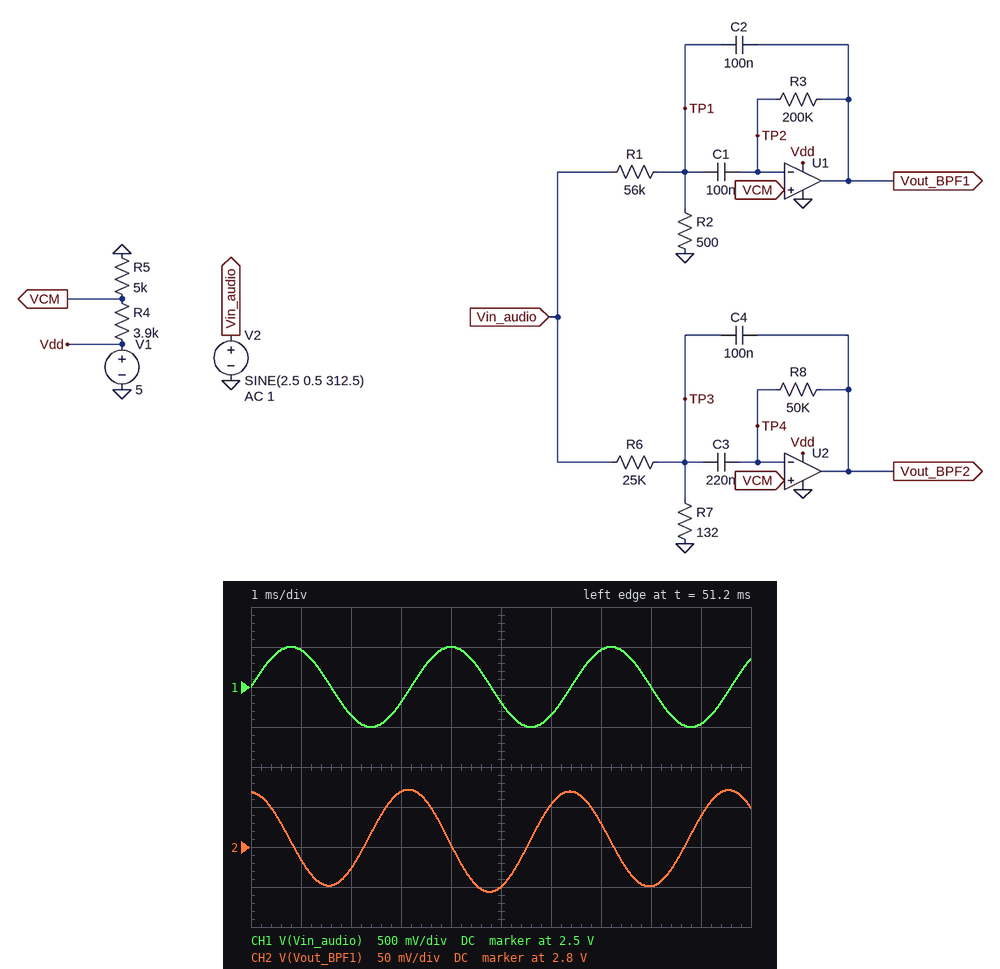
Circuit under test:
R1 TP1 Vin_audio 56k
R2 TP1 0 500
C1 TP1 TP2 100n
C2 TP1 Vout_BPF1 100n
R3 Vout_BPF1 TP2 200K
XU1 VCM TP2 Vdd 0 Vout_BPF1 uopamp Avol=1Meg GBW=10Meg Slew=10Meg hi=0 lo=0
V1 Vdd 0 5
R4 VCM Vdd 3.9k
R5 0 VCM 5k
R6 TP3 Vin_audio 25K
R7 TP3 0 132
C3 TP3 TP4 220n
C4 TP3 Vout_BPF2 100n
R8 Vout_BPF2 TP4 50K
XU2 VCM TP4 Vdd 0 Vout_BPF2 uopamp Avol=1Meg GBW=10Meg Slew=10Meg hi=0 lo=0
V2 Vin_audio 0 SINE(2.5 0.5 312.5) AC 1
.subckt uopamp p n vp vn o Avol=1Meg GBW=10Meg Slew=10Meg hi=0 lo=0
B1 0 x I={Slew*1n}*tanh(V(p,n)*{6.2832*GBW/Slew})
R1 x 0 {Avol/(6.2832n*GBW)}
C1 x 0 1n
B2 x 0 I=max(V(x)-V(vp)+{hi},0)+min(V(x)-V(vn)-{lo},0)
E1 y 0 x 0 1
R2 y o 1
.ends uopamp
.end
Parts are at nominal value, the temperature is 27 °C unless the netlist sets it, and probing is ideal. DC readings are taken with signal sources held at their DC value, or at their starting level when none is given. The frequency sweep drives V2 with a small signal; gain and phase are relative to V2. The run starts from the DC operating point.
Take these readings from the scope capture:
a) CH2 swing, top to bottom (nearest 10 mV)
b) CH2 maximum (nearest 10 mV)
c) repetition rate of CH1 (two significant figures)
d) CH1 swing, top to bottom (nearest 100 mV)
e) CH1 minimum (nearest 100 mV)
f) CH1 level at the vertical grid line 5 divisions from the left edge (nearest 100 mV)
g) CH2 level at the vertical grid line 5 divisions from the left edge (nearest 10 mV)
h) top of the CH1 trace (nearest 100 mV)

130 mV
2.87 V
310 Hz
1.0 V
2.0 V
2.3 V
2.75 V
3.0 V
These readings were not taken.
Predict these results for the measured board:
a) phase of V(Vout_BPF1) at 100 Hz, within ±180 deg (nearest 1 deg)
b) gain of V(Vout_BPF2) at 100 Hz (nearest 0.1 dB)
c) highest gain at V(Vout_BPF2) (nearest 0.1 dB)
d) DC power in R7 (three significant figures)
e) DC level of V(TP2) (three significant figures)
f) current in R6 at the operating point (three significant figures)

-96 deg
-28.3 dB
2.8 dB
1.31 µW
2.81 V
99.5 µA
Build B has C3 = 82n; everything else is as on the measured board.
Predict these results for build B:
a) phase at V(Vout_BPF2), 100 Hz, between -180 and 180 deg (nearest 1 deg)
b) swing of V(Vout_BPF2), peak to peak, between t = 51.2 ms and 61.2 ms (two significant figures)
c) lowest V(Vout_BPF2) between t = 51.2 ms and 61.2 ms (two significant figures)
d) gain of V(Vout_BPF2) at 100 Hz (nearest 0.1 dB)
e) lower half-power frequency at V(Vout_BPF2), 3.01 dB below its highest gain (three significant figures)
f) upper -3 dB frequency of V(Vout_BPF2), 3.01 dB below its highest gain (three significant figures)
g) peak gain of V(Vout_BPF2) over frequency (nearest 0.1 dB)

-91 deg
53 mV
2.8 V
-37.2 dB
651 Hz
722 Hz
-0.9 dB
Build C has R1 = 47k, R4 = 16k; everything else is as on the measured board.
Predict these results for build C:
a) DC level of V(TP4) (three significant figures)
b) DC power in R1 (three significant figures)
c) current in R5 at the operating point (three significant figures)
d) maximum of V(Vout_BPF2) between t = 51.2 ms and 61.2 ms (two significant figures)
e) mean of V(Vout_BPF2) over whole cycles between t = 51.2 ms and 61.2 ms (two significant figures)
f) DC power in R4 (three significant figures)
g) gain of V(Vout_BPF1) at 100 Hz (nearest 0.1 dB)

1.19 V
130 µW
238 µA
1.3 V
1.2 V
907 µW
-13.3 dB
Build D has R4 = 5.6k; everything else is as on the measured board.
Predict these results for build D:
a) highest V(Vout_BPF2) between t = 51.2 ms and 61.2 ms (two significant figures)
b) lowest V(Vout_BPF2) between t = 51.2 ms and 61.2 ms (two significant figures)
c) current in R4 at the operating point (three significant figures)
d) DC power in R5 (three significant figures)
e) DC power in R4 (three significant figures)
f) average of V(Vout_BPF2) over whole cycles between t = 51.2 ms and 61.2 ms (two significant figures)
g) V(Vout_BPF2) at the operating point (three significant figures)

2.5 V
2.2 V
472 µA
1.11 mW
1.25 mW
2.4 V
2.36 V
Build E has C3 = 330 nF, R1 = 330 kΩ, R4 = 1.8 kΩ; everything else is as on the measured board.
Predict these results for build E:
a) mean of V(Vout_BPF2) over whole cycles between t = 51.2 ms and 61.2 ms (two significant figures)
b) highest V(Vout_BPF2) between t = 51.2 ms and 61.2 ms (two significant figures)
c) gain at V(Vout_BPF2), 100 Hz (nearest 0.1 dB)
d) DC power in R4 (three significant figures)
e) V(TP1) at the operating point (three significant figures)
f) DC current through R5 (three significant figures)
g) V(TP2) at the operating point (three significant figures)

3.7 V
4.1 V
-24.5 dB
973 µW
3.78 mV
735 µA
3.68 V
